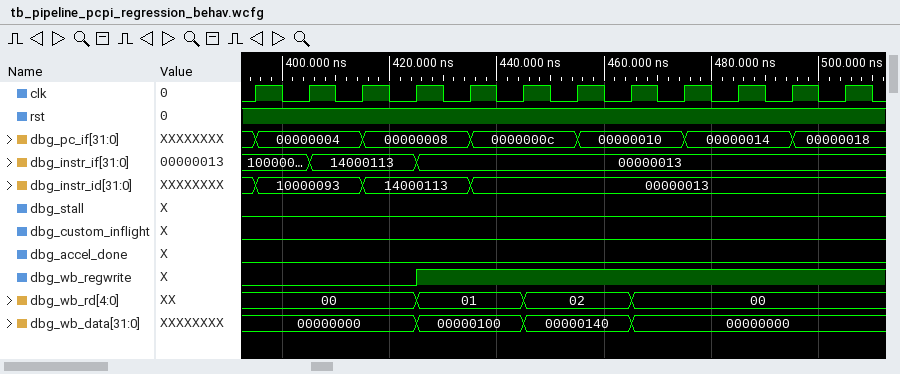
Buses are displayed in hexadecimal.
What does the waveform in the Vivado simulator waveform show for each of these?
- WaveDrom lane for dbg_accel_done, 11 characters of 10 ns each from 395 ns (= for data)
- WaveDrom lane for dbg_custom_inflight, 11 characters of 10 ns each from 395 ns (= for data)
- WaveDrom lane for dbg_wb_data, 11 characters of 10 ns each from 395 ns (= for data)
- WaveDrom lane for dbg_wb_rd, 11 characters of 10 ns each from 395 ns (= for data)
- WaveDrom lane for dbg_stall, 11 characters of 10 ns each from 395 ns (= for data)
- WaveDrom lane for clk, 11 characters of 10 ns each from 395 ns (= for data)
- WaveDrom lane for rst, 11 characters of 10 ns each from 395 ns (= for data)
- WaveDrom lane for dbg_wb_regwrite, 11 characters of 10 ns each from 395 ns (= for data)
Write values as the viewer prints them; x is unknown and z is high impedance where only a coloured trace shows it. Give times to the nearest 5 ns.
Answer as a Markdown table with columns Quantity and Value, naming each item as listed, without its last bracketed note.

| Quantity | Value |
|---|---|
| WaveDrom lane for dbg_accel_done, 11 characters of 10 ns each from 395 ns | {name: 'dbg_accel_done', wave: '0..........'} |
| WaveDrom lane for dbg_custom_inflight, 11 characters of 10 ns each from 395 ns | {name: 'dbg_custom_inflight', wave: '0..........'} |
| WaveDrom lane for dbg_wb_data, 11 characters of 10 ns each from 395 ns | {name: 'dbg_wb_data', wave: '=..=.=.=...', data: '00000000 00000100 00000140 00000000'} |
| WaveDrom lane for dbg_wb_rd, 11 characters of 10 ns each from 395 ns | {name: 'dbg_wb_rd', wave: '=..=.=.=...', data: '00 01 02 00'} |
| WaveDrom lane for dbg_stall, 11 characters of 10 ns each from 395 ns | {name: 'dbg_stall', wave: '0..........'} |
| WaveDrom lane for clk, 11 characters of 10 ns each from 395 ns | {name: 'clk', wave: 'p..........'} |
| WaveDrom lane for rst, 11 characters of 10 ns each from 395 ns | {name: 'rst', wave: '1..........'} |
| WaveDrom lane for dbg_wb_regwrite, 11 characters of 10 ns each from 395 ns | {name: 'dbg_wb_regwrite', wave: '0..1.......'} |
